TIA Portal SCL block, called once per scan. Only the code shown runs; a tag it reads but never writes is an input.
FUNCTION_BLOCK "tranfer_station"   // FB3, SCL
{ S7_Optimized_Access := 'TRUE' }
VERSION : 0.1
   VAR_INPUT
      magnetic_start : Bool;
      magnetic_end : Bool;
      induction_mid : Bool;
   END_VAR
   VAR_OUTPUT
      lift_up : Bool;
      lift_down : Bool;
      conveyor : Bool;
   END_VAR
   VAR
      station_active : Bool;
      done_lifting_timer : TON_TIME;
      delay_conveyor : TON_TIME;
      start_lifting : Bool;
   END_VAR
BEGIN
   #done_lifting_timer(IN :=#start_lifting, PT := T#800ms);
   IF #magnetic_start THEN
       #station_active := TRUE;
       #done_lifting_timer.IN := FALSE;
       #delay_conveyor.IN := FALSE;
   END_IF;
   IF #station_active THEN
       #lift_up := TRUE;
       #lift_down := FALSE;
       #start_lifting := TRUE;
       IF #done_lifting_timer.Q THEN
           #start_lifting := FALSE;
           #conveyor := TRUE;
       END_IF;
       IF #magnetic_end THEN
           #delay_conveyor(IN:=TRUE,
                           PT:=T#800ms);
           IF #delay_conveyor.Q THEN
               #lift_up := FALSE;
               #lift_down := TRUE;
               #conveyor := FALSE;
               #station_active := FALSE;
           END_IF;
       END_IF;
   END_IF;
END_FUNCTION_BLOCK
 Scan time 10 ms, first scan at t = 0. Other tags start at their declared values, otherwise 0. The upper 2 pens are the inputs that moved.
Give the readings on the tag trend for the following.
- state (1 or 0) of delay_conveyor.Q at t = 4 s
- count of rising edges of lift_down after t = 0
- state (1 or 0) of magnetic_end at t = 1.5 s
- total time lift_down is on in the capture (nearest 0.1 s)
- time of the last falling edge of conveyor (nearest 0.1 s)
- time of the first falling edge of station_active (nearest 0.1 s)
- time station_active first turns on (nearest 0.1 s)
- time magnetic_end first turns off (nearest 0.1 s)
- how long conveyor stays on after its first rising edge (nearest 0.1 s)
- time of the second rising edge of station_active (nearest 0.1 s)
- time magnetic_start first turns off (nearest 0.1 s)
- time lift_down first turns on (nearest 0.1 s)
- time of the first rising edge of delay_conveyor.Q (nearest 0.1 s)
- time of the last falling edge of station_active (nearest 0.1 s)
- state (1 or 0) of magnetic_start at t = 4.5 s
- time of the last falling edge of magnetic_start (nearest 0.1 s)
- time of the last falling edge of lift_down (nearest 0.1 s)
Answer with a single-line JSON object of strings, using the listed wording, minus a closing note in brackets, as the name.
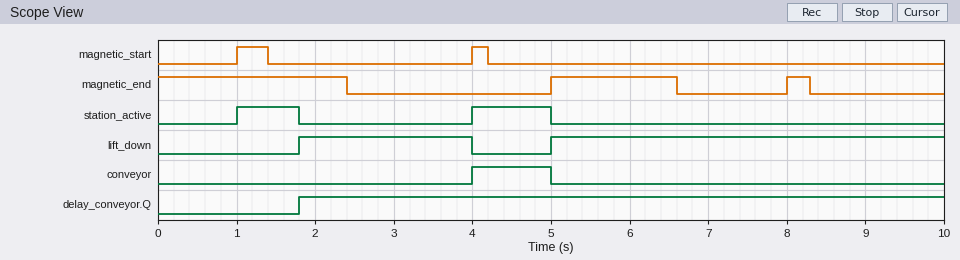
{"state (1 or 0) of delay_conveyor.Q at t = 4 s": "1", "count of rising edges of lift_down after t = 0": "2", "state (1 or 0) of magnetic_end at t = 1.5 s": "1", "total time lift_down is on in the capture": "7.2 s", "time of the last falling edge of conveyor": "5.0 s", "time of the first falling edge of station_active": "1.8 s", "time station_active first turns on": "1.0 s", "time magnetic_end first turns off": "2.4 s", "how long conveyor stays on after its first rising edge": "1.0 s", "time of the second rising edge of station_active": "4.0 s", "time magnetic_start first turns off": "1.4 s", "time lift_down first turns on": "1.8 s", "time of the first rising edge of delay_conveyor.Q": "1.8 s", "time of the last falling edge of station_active": "5.0 s", "state (1 or 0) of magnetic_start at t = 4.5 s": "0", "time of the last falling edge of magnetic_start": "4.2 s", "time of the last falling edge of lift_down": "4.0 s"}
